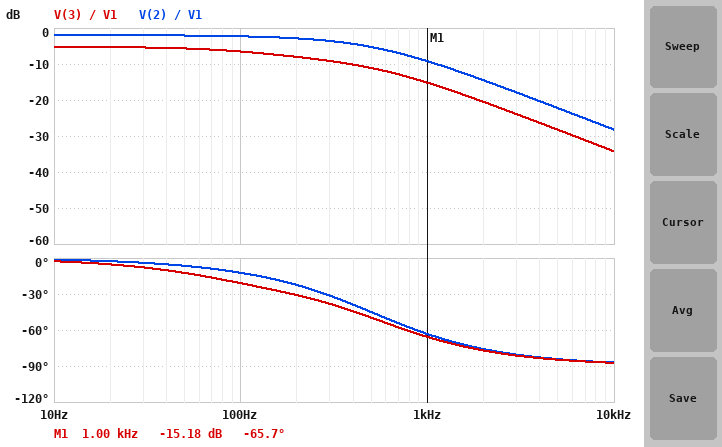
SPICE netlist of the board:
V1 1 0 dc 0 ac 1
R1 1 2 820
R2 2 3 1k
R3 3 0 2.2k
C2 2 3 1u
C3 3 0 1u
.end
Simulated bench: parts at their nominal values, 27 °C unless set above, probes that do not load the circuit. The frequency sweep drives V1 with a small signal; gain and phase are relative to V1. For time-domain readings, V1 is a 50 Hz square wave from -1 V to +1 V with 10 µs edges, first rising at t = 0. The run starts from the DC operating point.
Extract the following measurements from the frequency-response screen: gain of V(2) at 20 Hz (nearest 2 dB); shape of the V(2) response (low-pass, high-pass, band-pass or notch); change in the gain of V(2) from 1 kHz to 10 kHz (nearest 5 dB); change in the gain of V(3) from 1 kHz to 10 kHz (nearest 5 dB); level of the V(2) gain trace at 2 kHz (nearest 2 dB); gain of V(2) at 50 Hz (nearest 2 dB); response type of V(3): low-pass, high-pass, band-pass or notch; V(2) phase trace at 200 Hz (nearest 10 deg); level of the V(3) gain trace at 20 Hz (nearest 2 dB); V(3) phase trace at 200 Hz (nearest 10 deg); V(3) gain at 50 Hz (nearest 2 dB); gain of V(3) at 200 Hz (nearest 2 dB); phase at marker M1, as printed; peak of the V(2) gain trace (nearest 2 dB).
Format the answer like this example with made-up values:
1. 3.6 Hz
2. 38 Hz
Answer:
1. -2 dB
2. low-pass
3. -20 dB
4. -20 dB
5. -14 dB
6. -2 dB
7. low-pass
8. -20 deg
9. -6 dB
10. -30 deg
11. -6 dB
12. -8 dB
13. -65.7 deg
14. -2 dB
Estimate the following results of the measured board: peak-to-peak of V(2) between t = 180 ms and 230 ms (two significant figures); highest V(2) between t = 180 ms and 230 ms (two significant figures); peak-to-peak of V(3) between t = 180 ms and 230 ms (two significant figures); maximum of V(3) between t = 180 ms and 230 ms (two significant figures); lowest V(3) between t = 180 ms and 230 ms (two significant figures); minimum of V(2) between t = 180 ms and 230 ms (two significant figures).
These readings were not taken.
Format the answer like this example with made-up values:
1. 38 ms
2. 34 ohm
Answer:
1. 1.6 V
2. 800 mV
3. 1.1 V
4. 550 mV
5. -550 mV
6. -800 mV
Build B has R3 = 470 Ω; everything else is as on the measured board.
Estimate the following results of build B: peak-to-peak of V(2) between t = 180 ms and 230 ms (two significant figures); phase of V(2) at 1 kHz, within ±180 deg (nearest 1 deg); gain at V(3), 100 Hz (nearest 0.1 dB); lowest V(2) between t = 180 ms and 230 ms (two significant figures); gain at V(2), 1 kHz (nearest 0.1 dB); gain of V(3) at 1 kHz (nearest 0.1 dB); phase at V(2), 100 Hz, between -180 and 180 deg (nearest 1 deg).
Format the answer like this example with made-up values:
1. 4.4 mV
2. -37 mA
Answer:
1. 1.3 V
2. -58 deg
3. -13.2 dB
4. -640 mV
5. -9.7 dB
6. -15.9 dB
7. -10 deg
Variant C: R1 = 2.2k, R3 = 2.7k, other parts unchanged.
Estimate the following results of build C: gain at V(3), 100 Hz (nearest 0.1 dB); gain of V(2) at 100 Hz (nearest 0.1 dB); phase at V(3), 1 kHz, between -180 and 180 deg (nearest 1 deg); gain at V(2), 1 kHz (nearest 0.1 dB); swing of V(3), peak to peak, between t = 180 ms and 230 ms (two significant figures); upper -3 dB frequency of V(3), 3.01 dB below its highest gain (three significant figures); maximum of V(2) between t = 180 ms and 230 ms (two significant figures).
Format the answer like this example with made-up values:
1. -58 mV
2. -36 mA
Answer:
1. -9.2 dB
2. -5.3 dB
3. -79 deg
4. -17.1 dB
5. 910 mV
6. 118 Hz
7. 630 mV
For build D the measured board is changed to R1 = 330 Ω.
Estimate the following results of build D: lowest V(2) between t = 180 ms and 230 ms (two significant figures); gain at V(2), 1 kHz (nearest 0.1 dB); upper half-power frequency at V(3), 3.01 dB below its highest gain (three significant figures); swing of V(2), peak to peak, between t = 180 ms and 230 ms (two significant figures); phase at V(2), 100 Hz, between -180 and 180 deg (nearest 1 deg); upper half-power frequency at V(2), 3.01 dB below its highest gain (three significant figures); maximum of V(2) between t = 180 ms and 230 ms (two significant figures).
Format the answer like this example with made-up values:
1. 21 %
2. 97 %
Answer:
1. -910 mV
2. -3.7 dB
3. 361 Hz
4. 1.8 V
5. -6 deg
6. 1.05 kHz
7. 910 mV
